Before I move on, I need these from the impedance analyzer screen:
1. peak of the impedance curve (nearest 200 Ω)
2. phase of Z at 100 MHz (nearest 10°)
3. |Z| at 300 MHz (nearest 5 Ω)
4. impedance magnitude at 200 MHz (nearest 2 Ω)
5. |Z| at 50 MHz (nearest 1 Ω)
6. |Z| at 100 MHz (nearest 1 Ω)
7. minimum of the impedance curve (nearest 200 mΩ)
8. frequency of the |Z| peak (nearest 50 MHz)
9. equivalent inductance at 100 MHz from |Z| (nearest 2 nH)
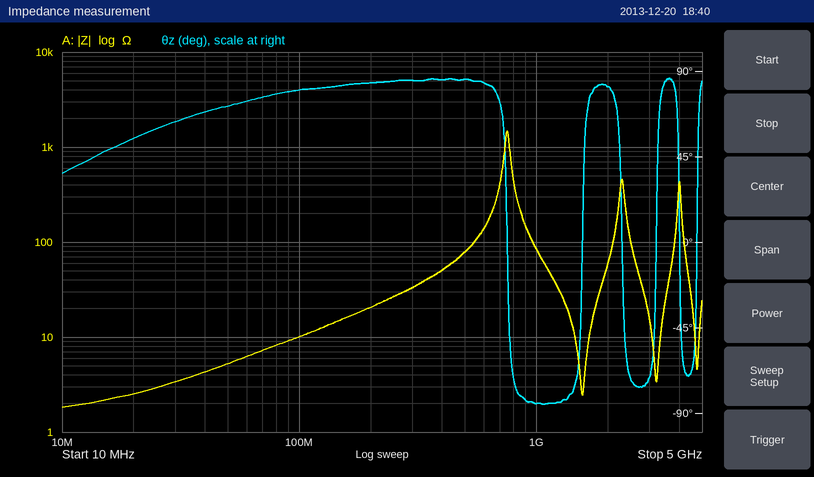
1.4 kΩ
80°
35 Ω
20 Ω
5 Ω
10 Ω
1.8 Ω
750 MHz
16 nH
